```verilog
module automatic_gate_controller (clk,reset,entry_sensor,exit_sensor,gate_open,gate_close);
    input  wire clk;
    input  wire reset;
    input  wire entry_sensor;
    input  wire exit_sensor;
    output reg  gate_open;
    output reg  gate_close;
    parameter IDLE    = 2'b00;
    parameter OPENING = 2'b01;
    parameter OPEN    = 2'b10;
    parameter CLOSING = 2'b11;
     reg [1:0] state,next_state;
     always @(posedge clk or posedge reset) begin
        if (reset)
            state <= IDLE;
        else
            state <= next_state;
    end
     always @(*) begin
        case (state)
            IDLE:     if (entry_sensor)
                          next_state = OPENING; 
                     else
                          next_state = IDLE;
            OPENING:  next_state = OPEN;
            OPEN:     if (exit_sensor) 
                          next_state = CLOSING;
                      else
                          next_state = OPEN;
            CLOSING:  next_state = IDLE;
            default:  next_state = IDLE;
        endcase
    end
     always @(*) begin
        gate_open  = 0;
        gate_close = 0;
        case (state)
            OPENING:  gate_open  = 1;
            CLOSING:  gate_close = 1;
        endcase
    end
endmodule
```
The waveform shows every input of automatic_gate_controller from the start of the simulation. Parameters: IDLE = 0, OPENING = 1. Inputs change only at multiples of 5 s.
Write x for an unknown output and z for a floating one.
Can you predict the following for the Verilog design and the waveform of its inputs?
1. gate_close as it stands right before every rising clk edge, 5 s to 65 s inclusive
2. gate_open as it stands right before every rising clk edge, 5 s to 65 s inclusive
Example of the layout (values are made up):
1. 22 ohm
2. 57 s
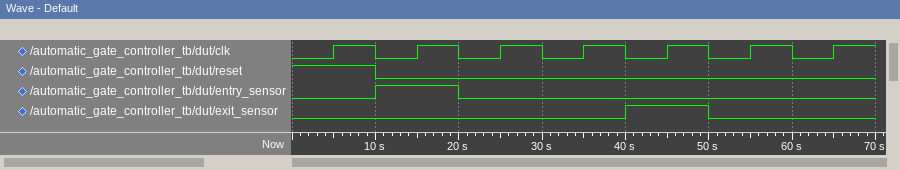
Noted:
1. 0 0 0 0 0 1 0
2. 0 0 1 0 0 0 0
